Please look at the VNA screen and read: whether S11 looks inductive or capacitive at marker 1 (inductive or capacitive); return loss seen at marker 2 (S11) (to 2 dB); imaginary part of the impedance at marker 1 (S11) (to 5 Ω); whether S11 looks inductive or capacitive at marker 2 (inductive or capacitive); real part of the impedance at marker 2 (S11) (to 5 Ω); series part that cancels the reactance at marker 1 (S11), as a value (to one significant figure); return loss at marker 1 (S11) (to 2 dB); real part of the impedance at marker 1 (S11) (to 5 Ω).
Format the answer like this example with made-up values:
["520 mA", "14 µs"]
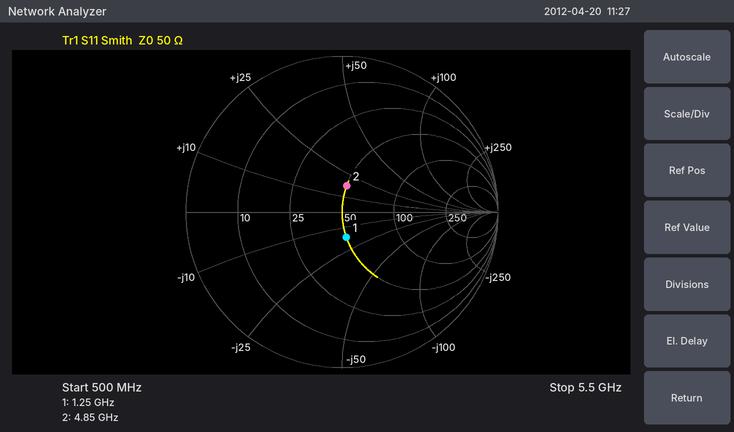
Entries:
["capacitive", "16 dB", "-15 Ω", "inductive", "50 Ω", "2 nH", "16 dB", "50 Ω"]
